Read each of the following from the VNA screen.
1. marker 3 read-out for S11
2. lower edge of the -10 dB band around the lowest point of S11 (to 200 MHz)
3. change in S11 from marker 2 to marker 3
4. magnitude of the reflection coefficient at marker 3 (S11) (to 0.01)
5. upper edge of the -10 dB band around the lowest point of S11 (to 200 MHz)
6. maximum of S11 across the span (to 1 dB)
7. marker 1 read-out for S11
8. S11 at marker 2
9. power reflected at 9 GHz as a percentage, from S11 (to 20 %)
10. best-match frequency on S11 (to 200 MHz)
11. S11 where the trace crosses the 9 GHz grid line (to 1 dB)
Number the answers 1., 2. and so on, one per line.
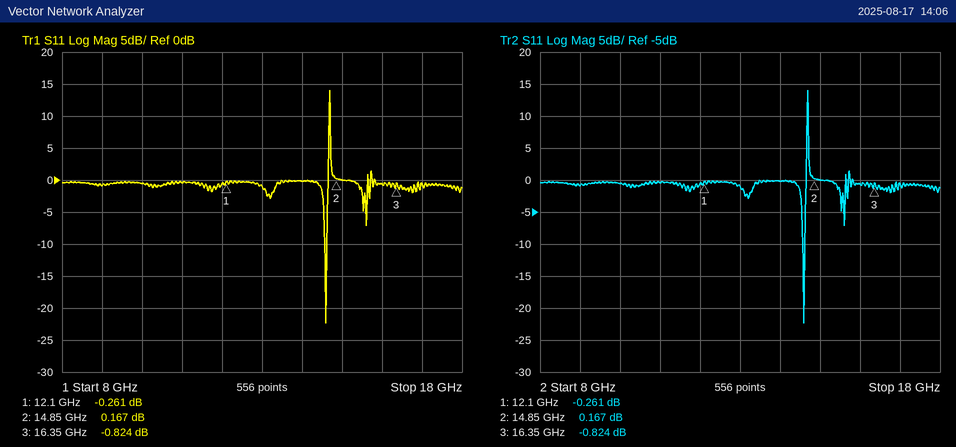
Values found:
1. -0.824 dB
2. 14.6 GHz
3. -0.991 dB
4. 0.91
5. 14.6 GHz
6. 14 dB
7. -0.261 dB
8. 0.167 dB
9. 80 %
10. 14.6 GHz
11. -1 dB
